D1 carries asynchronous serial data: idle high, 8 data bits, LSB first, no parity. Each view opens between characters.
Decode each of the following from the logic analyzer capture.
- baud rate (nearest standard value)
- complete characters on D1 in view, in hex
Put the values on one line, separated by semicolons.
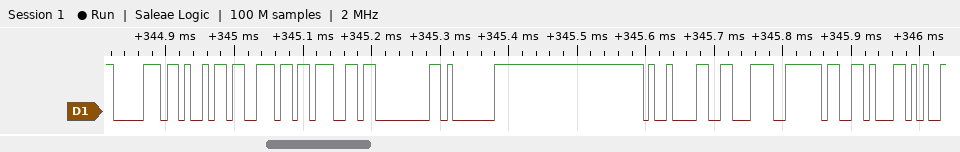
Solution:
115200 baud; 70, 69, 6E, 67, 00, 01, 09, C6, 7E, 16
